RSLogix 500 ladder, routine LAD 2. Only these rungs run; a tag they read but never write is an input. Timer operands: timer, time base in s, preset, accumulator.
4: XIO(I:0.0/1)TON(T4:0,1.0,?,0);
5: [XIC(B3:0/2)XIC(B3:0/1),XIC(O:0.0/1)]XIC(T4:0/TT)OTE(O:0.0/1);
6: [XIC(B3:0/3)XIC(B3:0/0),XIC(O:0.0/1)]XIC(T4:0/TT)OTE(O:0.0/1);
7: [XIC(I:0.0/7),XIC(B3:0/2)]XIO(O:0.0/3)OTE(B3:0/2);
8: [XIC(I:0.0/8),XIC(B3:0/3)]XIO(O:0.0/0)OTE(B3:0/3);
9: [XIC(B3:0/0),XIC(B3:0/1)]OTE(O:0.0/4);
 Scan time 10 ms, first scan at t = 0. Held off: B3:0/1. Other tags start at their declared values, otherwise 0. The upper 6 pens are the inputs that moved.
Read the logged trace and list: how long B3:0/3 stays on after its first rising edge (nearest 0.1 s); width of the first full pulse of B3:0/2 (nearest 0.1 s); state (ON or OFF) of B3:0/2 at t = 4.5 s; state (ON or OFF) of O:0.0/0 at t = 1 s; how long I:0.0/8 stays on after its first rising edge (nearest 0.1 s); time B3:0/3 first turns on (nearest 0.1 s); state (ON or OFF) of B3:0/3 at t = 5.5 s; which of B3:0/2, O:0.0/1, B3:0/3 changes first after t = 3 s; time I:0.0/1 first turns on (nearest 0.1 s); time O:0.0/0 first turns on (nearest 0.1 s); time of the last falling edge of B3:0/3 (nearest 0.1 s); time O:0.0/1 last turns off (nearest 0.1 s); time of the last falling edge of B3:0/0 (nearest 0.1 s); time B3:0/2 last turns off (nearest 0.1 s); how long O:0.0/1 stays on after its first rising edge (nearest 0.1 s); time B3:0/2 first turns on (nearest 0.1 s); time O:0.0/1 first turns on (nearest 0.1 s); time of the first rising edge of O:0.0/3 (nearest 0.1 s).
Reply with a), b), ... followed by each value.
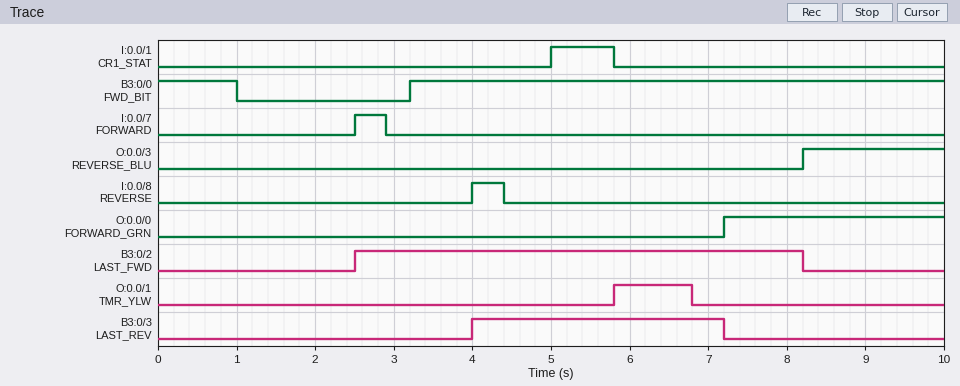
a) 3.2 s
b) 5.7 s
c) ON
d) OFF
e) 0.4 s
f) 4.0 s
g) ON
h) B3:0/3
i) 5.0 s
j) 7.2 s
k) 7.2 s
l) 6.8 s
m) 1.0 s
n) 8.2 s
o) 1.0 s
p) 2.5 s
q) 5.8 s
r) 8.2 s
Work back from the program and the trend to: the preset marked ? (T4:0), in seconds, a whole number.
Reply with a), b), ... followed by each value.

a) 1 s
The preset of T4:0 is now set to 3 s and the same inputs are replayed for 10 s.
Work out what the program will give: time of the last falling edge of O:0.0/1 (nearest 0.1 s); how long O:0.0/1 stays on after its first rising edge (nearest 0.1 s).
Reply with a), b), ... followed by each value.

a) 8.8 s
b) 3.0 s
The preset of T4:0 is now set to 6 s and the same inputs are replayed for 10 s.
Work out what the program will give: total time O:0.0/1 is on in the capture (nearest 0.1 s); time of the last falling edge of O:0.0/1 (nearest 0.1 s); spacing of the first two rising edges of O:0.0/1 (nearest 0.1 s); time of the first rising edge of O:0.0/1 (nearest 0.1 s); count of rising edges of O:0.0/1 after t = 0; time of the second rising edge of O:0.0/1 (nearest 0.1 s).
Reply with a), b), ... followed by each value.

a) 5.2 s
b) 5.0 s
c) 1.8 s
d) 4.0 s
e) 2
f) 5.8 s
